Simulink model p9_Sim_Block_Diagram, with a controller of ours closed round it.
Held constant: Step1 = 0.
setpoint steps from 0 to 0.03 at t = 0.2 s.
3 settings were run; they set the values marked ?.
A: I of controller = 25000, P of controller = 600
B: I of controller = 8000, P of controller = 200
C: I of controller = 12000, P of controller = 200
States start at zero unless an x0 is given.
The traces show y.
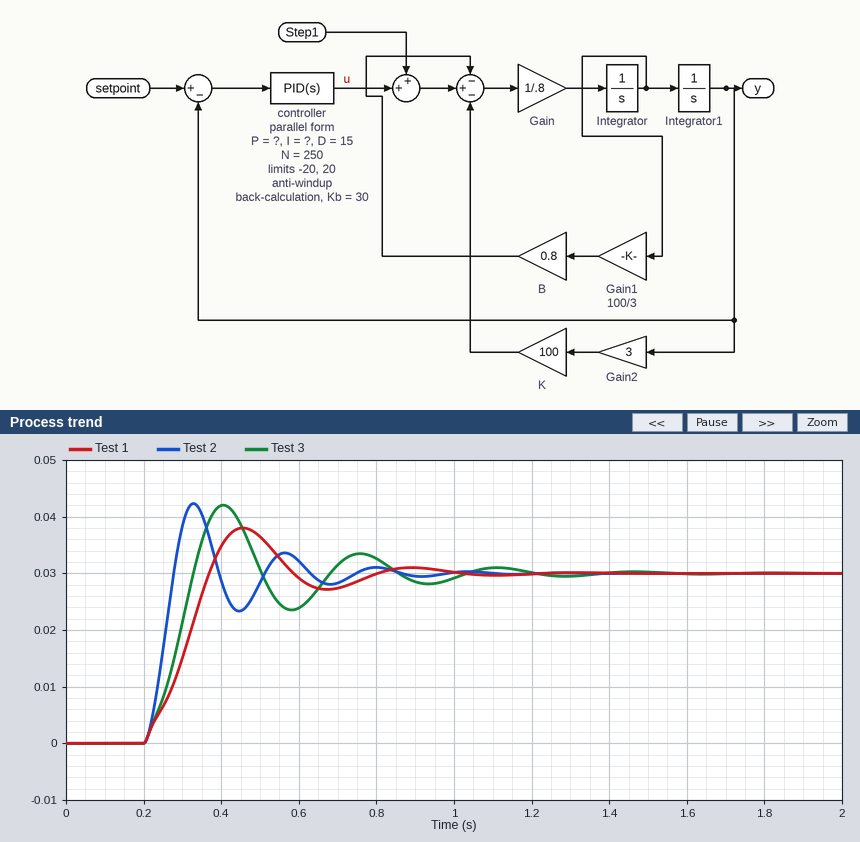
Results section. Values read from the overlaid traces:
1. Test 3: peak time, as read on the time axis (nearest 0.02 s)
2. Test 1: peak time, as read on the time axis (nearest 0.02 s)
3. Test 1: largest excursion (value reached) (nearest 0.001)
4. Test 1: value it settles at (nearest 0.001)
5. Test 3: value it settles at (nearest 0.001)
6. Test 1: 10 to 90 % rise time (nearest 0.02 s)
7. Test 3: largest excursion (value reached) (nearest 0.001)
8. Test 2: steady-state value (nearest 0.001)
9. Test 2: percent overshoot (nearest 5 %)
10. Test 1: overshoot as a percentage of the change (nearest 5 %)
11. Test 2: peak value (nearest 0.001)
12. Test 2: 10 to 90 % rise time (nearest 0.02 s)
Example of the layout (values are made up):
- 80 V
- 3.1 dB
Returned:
- 0.40 s
- 0.46 s
- 0.038
- 0.030
- 0.030
- 0.14 s
- 0.042
- 0.030
- 40 %
- 25 %
- 0.042
- 0.06 s
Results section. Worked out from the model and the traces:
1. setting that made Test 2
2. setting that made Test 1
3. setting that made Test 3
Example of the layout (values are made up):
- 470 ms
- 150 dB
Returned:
- A
- B
- C
